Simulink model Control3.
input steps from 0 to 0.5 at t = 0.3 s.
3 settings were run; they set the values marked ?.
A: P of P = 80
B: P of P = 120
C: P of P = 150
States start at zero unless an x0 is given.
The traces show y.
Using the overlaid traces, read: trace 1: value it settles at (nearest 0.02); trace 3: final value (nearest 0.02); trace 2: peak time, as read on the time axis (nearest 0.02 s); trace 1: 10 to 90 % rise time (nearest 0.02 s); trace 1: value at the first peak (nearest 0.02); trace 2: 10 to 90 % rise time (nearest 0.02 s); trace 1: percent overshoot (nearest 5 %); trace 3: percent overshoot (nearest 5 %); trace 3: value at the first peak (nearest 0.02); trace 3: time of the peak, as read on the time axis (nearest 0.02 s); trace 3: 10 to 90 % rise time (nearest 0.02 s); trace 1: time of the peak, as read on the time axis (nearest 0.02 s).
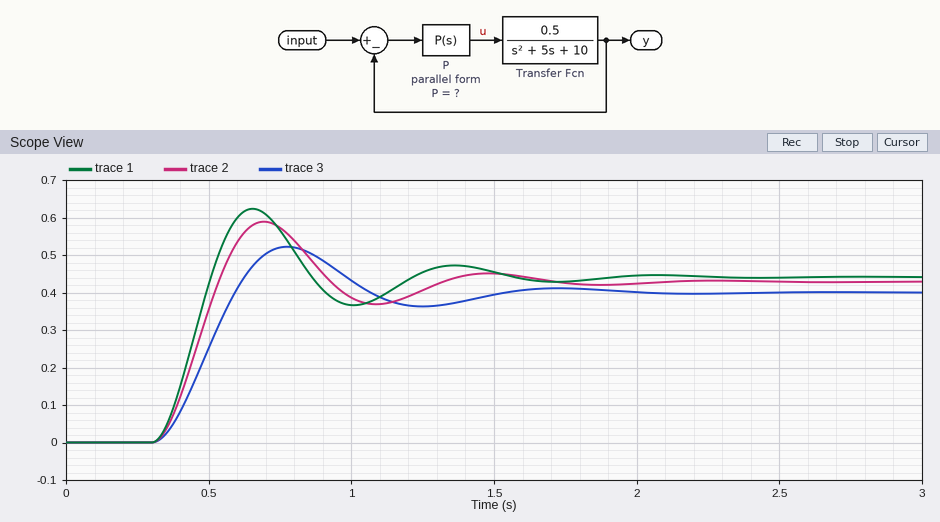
0.44
0.40
0.70 s
0.14 s
0.62
0.16 s
40 %
30 %
0.52
0.78 s
0.20 s
0.66 s
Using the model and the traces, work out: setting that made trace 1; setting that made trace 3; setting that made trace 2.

C
A
B
